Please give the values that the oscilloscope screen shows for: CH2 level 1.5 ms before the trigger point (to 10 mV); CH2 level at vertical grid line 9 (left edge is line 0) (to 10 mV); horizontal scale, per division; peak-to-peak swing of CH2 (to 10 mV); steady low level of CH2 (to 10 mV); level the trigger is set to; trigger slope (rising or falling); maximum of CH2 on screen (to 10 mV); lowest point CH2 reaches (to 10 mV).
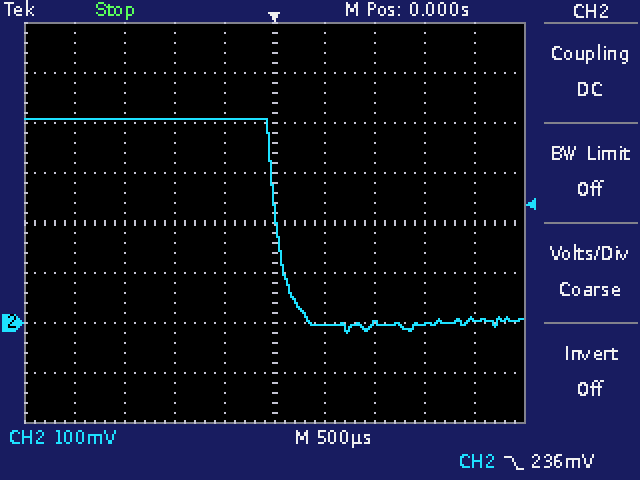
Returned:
410 mV
10 mV
500 µs
430 mV
0 mV
236 mV
falling
410 mV
-20 mV
